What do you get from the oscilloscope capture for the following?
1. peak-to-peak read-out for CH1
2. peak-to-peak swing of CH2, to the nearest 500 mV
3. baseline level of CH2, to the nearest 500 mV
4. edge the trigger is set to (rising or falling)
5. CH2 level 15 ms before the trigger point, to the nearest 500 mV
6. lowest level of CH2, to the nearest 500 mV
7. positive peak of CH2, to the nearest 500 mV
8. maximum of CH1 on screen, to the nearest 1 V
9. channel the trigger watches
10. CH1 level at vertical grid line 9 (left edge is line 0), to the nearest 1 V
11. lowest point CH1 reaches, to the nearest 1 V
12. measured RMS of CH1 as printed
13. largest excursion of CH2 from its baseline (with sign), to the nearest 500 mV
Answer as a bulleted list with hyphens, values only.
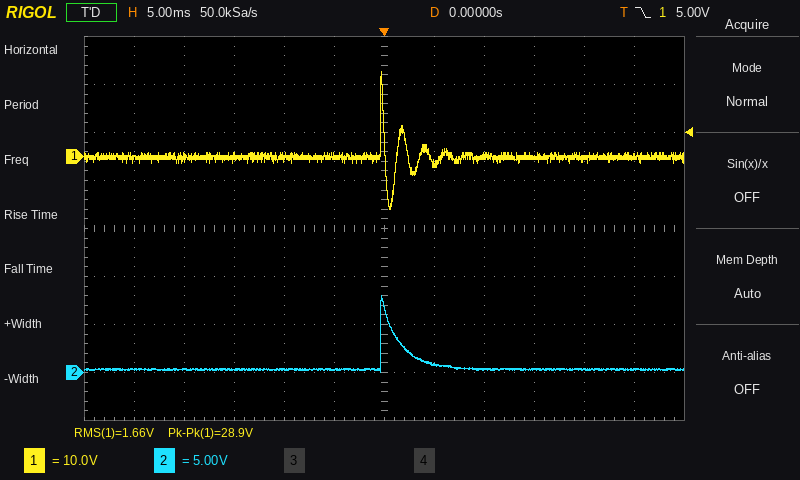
- 28.9 V
- 8.0 V
- 500 mV
- falling
- 500 mV
- 0.0 V
- 8.0 V
- 18 V
- CH1
- 0 V
- -11 V
- 1.66 V
- +7.5 V
